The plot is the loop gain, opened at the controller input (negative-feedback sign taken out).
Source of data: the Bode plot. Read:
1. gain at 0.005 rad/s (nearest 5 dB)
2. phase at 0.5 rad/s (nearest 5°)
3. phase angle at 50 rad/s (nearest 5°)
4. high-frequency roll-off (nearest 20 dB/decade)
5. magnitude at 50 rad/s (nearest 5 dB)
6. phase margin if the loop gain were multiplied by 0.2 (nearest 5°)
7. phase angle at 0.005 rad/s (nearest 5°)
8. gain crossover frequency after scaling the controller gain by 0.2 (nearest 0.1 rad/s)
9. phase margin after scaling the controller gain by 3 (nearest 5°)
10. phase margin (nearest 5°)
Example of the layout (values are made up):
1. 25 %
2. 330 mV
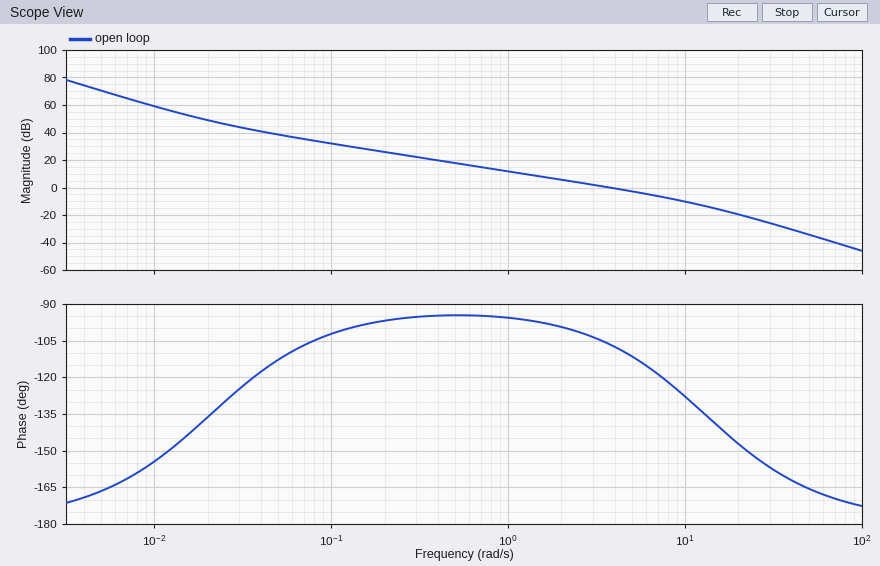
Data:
1. 70 dB
2. -95°
3. -165°
4. -40 dB/decade
5. -35 dB
6. 85°
7. -165°
8. 0.8 rad/s
9. 55°
10. 75°
